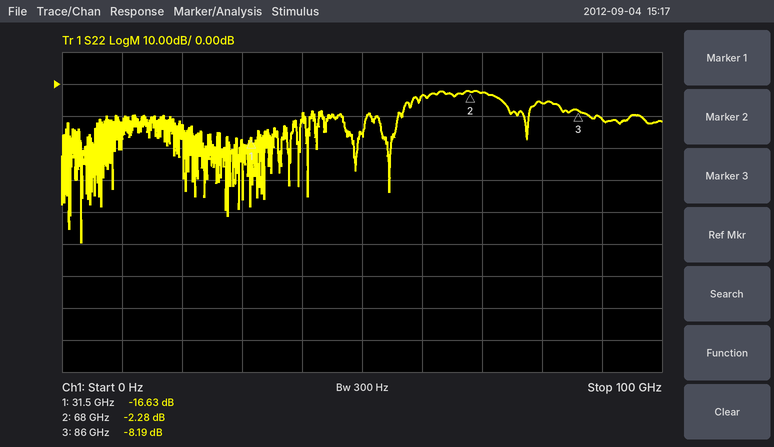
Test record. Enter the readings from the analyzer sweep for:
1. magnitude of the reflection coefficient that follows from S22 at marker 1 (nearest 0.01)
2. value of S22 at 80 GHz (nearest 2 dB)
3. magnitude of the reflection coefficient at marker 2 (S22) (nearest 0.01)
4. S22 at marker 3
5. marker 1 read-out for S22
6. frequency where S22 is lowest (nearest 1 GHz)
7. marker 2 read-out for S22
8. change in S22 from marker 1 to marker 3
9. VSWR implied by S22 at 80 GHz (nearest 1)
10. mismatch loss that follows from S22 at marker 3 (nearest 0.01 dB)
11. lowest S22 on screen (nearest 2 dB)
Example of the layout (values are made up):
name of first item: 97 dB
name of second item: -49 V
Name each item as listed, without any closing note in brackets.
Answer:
magnitude of the reflection coefficient that follows from S22 at marker 1: 0.15
value of S22 at 80 GHz: -6 dB
magnitude of the reflection coefficient at marker 2 (S22): 0.77
S22 at marker 3: -8.19 dB
marker 1 read-out for S22: -16.63 dB
frequency where S22 is lowest: 3 GHz
marker 2 read-out for S22: -2.28 dB
change in S22 from marker 1 to marker 3: 8.44 dB
VSWR implied by S22 at 80 GHz: 3
mismatch loss that follows from S22 at marker 3: 0.71 dB
lowest S22 on screen: -50 dB
